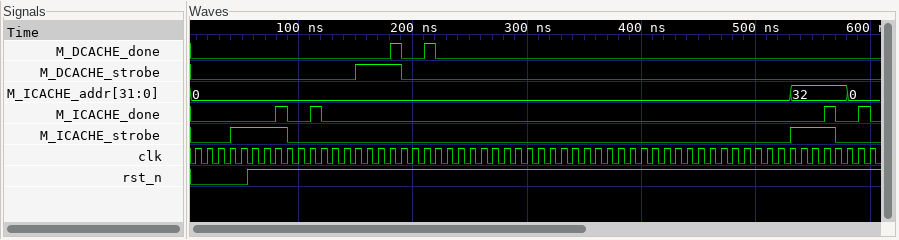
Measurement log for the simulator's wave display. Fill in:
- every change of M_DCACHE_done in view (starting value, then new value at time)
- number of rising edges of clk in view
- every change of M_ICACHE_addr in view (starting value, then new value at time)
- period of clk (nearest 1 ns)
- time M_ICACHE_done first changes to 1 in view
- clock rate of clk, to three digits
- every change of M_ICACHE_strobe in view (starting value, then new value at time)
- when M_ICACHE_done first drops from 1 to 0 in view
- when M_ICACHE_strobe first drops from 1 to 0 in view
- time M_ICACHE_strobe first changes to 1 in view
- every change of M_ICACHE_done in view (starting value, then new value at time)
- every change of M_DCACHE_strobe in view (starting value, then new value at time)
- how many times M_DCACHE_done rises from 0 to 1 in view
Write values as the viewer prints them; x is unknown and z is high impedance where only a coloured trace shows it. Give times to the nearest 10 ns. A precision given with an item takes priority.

0, 1 at 180 ns, 0 at 190 ns, 1 at 210 ns, 0 at 220 ns
60
0, 32 at 530 ns, 0 at 580 ns
10 ns
80 ns
100 MHz
0, 1 at 40 ns, 0 at 90 ns, 1 at 530 ns, 0 at 570 ns
90 ns
90 ns
40 ns
0, 1 at 80 ns, 0 at 90 ns, 1 at 110 ns, 0 at 120 ns, 1 at 560 ns, 0 at 570 ns, 1 at 590 ns, 0 at 600 ns
0, 1 at 150 ns, 0 at 190 ns
2
